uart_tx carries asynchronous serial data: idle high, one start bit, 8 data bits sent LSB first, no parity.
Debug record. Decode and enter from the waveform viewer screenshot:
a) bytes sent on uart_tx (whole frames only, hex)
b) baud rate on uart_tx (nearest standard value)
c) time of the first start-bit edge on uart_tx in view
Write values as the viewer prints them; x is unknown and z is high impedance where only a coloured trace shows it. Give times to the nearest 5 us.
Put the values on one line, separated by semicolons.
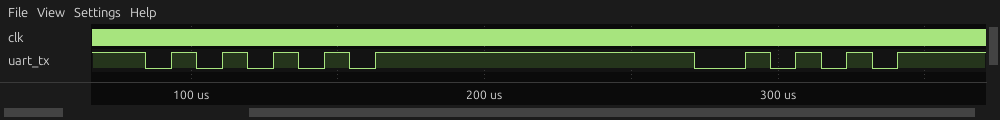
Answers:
55, AA; 115200 baud; 85 us
